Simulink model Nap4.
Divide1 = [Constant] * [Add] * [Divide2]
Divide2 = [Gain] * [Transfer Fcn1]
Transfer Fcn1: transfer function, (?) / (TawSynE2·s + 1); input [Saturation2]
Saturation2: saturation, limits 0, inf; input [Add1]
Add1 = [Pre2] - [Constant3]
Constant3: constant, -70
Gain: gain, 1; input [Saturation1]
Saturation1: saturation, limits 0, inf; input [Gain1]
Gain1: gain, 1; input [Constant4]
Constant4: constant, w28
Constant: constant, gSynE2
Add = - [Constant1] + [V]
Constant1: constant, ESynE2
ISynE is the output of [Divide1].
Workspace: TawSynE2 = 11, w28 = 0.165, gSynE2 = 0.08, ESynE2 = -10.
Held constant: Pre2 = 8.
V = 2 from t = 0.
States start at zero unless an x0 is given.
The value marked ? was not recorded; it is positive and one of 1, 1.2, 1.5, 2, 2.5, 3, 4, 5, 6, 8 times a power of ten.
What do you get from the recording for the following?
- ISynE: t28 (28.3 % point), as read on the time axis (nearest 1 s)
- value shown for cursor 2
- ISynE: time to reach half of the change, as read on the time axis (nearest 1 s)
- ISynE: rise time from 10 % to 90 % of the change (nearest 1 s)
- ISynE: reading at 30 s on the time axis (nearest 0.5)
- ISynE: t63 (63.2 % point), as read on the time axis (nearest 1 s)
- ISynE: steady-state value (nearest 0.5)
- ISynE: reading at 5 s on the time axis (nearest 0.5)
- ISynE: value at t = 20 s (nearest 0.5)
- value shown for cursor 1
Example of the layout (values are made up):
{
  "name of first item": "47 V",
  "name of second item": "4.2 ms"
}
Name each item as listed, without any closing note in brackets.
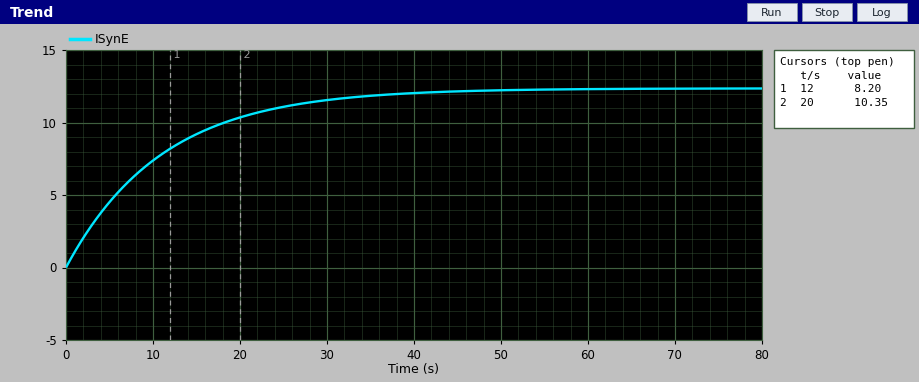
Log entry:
{
  "ISynE: t28 (28.3 % point), as read on the time axis": "4 s",
  "value shown for cursor 2": "10.35",
  "ISynE: time to reach half of the change, as read on the time axis": "8 s",
  "ISynE: rise time from 10 % to 90 % of the change": "24 s",
  "ISynE: reading at 30 s on the time axis": "11.5",
  "ISynE: t63 (63.2 % point), as read on the time axis": "11 s",
  "ISynE: steady-state value": "12.5",
  "ISynE: reading at 5 s on the time axis": "4.5",
  "ISynE: value at t = 20 s": "10.5",
  "value shown for cursor 1": "8.20"
}
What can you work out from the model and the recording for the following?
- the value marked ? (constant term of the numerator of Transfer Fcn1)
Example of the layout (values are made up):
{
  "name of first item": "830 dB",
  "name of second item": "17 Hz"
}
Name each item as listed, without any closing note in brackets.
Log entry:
{
  "the value marked ?": "1"
}
